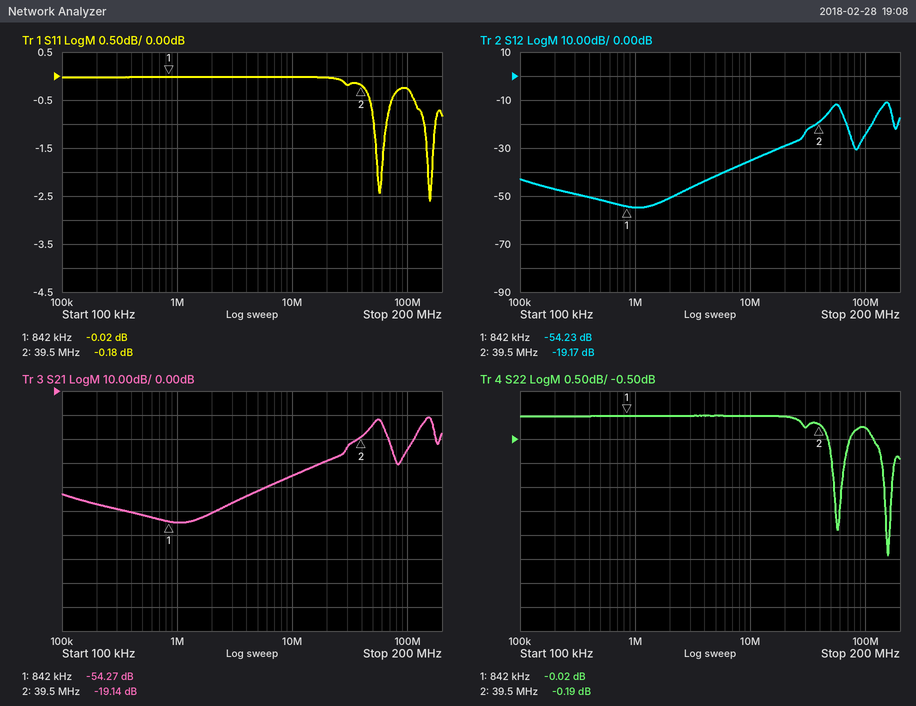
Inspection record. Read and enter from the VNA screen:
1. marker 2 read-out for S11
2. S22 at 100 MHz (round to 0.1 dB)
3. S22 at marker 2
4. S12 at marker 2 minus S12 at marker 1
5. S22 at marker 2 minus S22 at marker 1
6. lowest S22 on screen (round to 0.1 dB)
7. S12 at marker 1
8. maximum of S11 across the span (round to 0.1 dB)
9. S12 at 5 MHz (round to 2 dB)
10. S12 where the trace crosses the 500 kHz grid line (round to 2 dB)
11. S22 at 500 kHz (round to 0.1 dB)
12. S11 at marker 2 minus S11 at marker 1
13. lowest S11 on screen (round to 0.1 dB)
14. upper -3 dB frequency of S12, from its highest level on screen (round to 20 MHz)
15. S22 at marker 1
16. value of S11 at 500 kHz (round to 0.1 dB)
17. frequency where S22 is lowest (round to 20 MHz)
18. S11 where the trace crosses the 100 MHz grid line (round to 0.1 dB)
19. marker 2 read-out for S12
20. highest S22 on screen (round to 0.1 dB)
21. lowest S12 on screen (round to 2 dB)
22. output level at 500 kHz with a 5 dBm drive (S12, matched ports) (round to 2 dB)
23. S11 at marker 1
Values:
-0.18 dB
-0.3 dB
-0.19 dB
35.06 dB
-0.17 dB
-2.9 dB
-54.23 dB
0.0 dB
-42 dB
-52 dB
0.0 dB
-0.16 dB
-2.6 dB
160 MHz
-0.02 dB
0.0 dB
160 MHz
-0.3 dB
-19.17 dB
0.0 dB
-54 dB
-46 dBm
-0.02 dB
